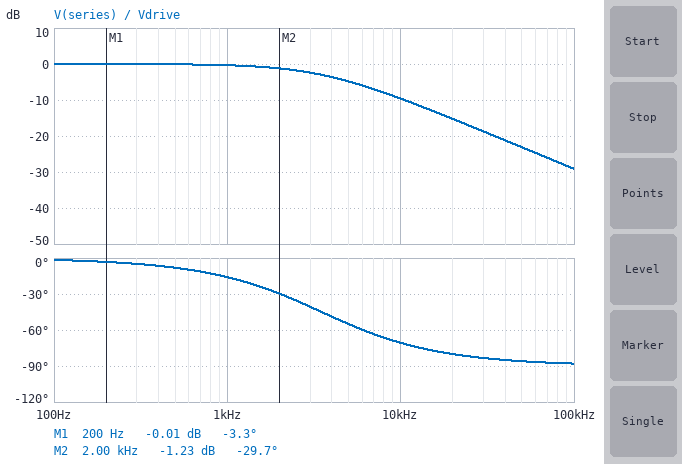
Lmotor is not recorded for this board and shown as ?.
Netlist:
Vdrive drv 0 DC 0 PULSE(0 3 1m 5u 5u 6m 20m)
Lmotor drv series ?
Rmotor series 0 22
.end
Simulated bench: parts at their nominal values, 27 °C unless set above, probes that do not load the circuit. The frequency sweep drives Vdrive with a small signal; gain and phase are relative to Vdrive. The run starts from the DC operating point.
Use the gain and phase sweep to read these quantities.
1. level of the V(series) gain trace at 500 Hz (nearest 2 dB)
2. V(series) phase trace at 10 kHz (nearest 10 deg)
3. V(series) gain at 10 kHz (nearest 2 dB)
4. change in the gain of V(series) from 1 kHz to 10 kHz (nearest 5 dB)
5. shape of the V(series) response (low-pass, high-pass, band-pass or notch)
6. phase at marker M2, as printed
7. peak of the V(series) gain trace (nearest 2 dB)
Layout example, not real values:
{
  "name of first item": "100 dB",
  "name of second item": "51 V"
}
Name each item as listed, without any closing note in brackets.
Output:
{
  "level of the V(series) gain trace at 500 Hz": "0 dB",
  "V(series) phase trace at 10 kHz": "-70 deg",
  "V(series) gain at 10 kHz": "-10 dB",
  "change in the gain of V(series) from 1 kHz to 10 kHz": "-10 dB",
  "shape of the V(series) response": "low-pass",
  "phase at marker M2, as printed": "-29.7 deg",
  "peak of the V(series) gain trace": "0 dB"
}
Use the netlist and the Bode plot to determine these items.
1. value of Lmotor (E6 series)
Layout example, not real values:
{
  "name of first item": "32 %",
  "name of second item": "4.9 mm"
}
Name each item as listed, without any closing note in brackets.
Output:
{
  "value of Lmotor": "1 mH"
}
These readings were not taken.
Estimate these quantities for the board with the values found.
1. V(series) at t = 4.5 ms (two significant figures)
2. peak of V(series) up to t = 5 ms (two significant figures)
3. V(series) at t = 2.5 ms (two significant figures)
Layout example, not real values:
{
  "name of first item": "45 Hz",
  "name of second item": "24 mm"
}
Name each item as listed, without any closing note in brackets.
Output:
{
  "V(series) at t = 4.5 ms": "3.0 V",
  "peak of V(series) up to t = 5 ms": "3.0 V",
  "V(series) at t = 2.5 ms": "3.0 V"
}
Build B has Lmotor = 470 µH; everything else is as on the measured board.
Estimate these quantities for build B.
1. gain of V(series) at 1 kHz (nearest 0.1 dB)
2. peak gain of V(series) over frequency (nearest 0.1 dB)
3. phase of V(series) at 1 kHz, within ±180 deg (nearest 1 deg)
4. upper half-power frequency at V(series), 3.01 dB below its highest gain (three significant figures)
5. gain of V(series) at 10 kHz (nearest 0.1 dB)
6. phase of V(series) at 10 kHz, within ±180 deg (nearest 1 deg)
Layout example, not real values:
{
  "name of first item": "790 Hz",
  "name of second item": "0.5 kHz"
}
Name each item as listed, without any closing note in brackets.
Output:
{
  "gain of V(series) at 1 kHz": "-0.1 dB",
  "peak gain of V(series) over frequency": "0 dB",
  "phase of V(series) at 1 kHz, within ±180 deg": "-8 deg",
  "upper half-power frequency at V(series), 3.01 dB below its highest gain": "7.45 kHz",
  "gain of V(series) at 10 kHz": "-4.5 dB",
  "phase of V(series) at 10 kHz, within ±180 deg": "-53 deg"
}
